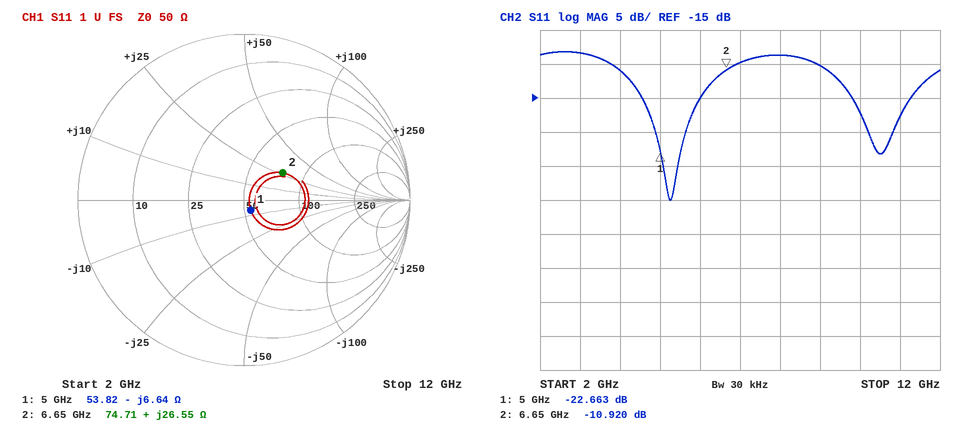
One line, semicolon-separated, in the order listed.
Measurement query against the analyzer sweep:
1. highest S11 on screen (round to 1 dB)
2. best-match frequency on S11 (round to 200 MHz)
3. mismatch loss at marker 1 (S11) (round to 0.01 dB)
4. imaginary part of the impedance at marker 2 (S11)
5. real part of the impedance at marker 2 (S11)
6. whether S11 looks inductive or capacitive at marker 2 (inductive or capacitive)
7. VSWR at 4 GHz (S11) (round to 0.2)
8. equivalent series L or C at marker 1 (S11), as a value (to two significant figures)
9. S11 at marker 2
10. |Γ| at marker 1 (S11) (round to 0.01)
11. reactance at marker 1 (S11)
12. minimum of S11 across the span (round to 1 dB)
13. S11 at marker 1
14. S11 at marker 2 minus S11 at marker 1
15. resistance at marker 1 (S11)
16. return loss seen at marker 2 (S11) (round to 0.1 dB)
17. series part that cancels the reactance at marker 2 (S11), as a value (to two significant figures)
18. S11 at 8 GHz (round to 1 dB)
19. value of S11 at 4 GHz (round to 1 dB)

-8 dB; 5.2 GHz; 0.02 dB; +26.55 Ω; 74.71 Ω; inductive; 1.8; 4.8 pF; -10.920 dB; 0.07; -6.64 Ω; -30 dB; -22.663 dB; 11.743 dB; 53.82 Ω; 10.9 dB; 900 fF; -9 dB; -11 dB
